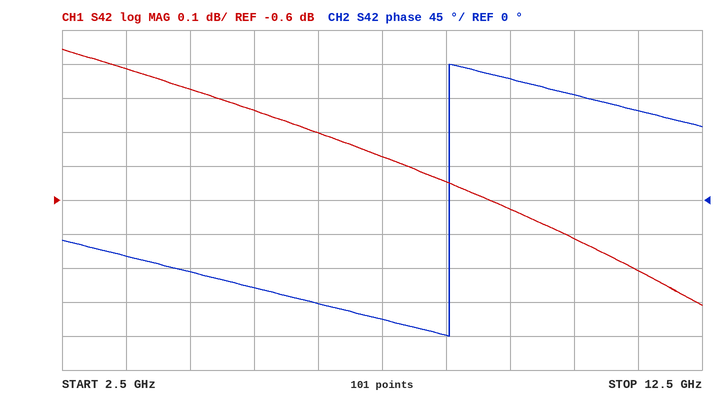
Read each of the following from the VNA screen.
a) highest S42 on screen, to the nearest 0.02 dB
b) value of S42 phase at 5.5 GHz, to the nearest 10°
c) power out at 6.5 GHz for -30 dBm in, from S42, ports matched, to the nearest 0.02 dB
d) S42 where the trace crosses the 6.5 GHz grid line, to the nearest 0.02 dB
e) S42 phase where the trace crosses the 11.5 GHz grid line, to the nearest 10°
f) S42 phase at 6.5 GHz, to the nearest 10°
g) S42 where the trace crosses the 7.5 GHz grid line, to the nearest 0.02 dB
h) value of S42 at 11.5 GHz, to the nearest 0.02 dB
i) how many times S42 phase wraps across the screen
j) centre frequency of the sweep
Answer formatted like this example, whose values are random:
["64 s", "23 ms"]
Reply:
["-0.16 dB", "-120°", "-30.40 dBm", "-0.40 dB", "120°", "-140°", "-0.48 dB", "-0.80 dB", "1", "7.5 GHz"]
